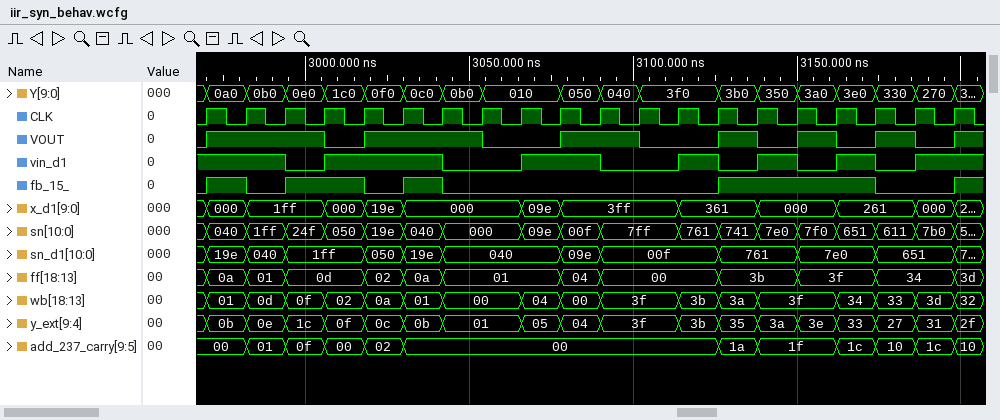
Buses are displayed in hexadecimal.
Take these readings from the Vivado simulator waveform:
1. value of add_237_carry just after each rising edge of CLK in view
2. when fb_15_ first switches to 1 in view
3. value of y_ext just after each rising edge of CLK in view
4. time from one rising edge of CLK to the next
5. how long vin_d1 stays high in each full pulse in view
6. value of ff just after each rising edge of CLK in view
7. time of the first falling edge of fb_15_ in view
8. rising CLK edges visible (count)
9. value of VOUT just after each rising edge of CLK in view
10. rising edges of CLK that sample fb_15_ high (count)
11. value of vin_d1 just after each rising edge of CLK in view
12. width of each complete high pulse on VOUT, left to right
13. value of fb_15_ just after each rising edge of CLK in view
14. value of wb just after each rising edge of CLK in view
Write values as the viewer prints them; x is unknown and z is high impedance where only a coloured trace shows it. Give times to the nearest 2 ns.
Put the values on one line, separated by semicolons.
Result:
00, 01, 0f, 00, 02, 00, 00, 00, 00, 00, 00, 00, 00, 1a, 1f, 1f, 1c, 10, 1c, 10; 2970 ns; 0b, 0e, 1c, 0f, 0c, 0b, 01, 01, 05, 04, 3f, 3f, 3b, 35, 3a, 3e, 33, 27, 31, 2f; 12 ns; 36 ns, 24 ns, 12 ns, 12 ns, 12 ns; 0a, 01, 0d, 0d, 02, 0a, 01, 01, 01, 04, 00, 00, 00, 3b, 3b, 3f, 3f, 34, 34, 3d; 2982 ns; 20; 1 1 1 0 1 1 1 0 0 1 1 0 0 1 0 1 0 1 0 1; 8; 1 1 0 1 1 1 0 0 1 1 0 0 1 0 1 0 1 0 1 1; 36 ns, 36 ns, 24 ns, 12 ns, 12 ns, 12 ns; 1 0 1 1 0 1 0 0 0 0 0 0 0 1 1 1 1 0 0 1; 01, 0d, 0f, 02, 0a, 01, 00, 00, 04, 00, 3f, 3f, 3b, 3a, 3f, 3f, 34, 33, 3d, 32
